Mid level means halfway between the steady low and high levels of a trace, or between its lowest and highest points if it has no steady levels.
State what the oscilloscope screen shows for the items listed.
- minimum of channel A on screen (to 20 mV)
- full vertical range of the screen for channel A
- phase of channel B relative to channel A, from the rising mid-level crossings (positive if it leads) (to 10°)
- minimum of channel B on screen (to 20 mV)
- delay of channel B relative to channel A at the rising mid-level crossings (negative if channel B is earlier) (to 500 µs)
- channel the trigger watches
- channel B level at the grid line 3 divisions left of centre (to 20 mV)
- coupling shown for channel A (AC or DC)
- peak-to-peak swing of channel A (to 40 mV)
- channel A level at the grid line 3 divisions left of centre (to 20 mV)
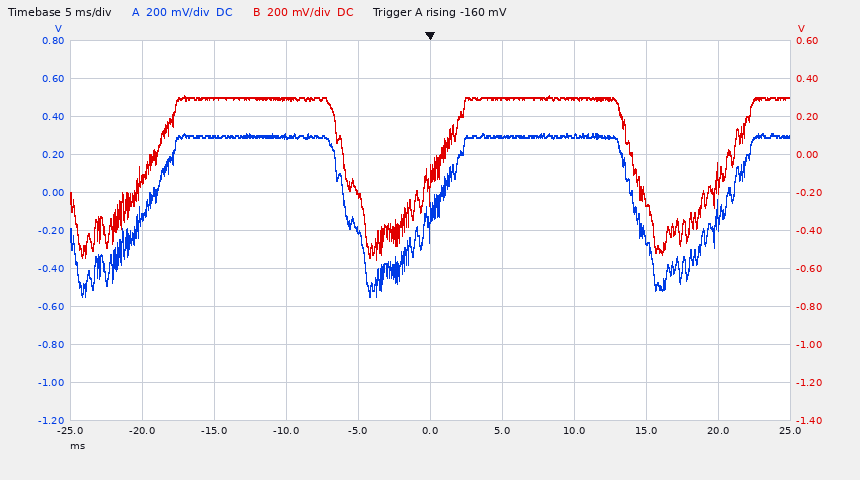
-540 mV
2 V
0°
-560 mV
0.0 ms
channel A
300 mV
DC
840 mV
300 mV
